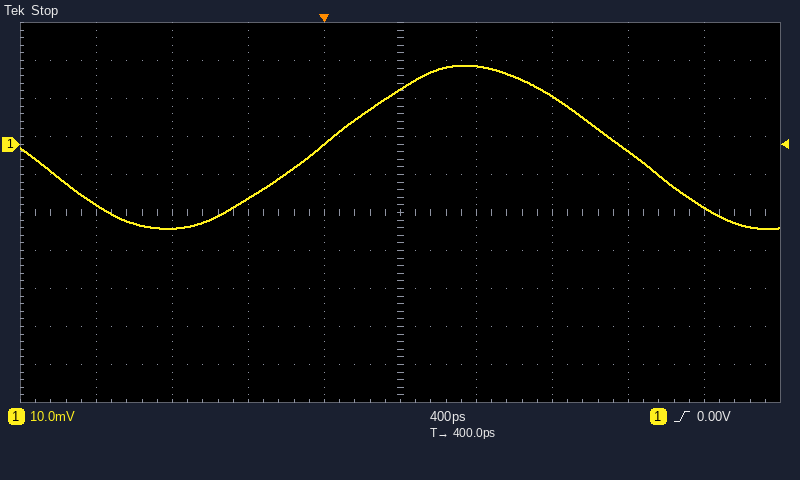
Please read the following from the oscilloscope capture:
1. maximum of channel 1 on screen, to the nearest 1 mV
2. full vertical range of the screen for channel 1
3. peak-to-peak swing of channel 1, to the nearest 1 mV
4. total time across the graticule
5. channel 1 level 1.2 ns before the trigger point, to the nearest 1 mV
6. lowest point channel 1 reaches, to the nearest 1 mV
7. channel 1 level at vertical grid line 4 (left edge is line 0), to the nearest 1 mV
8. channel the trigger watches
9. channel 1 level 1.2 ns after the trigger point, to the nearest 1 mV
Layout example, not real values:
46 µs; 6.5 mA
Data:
21 mV; 100 mV; 43 mV; 4 ns; -16 mV; -22 mV; 0 mV; channel 1; 13 mV
